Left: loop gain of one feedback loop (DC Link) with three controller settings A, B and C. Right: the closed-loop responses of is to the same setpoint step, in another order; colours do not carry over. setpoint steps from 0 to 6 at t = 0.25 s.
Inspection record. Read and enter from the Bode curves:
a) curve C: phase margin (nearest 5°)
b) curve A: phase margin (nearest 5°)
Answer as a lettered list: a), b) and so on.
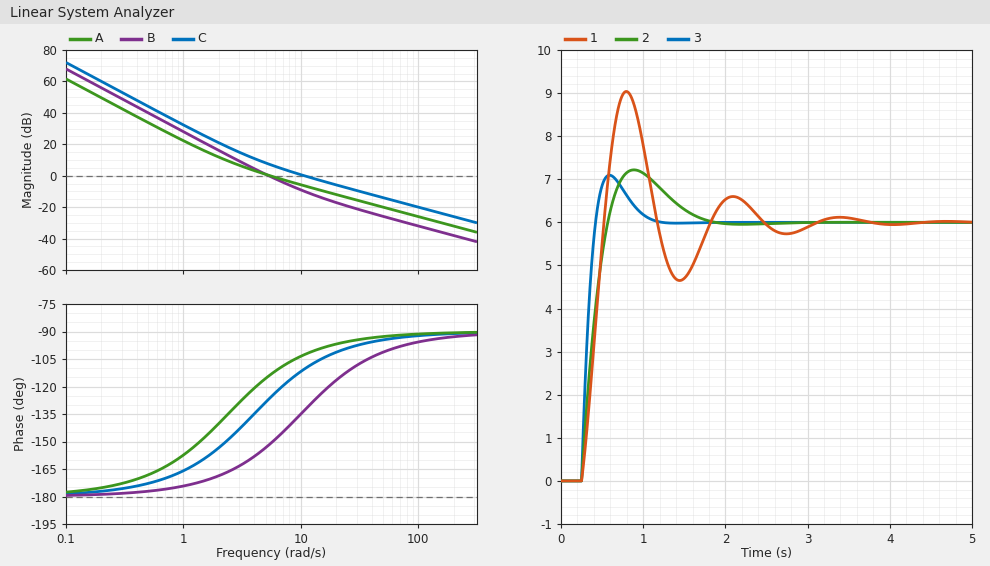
a) 70°
b) 65°
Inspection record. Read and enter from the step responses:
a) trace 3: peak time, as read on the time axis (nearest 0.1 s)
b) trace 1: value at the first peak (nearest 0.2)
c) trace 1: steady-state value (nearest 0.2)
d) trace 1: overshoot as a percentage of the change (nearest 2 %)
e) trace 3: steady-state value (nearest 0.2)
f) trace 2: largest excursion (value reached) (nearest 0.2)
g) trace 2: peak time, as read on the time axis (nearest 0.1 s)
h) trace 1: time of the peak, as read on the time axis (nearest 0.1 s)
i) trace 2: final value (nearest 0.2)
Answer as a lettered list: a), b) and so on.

a) 0.6 s
b) 9.0
c) 6.0
d) 50 %
e) 6.0
f) 7.2
g) 0.9 s
h) 0.8 s
i) 6.0
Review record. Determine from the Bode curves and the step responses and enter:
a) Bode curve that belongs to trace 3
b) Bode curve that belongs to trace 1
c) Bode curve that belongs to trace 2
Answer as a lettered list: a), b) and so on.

a) C
b) B
c) A
